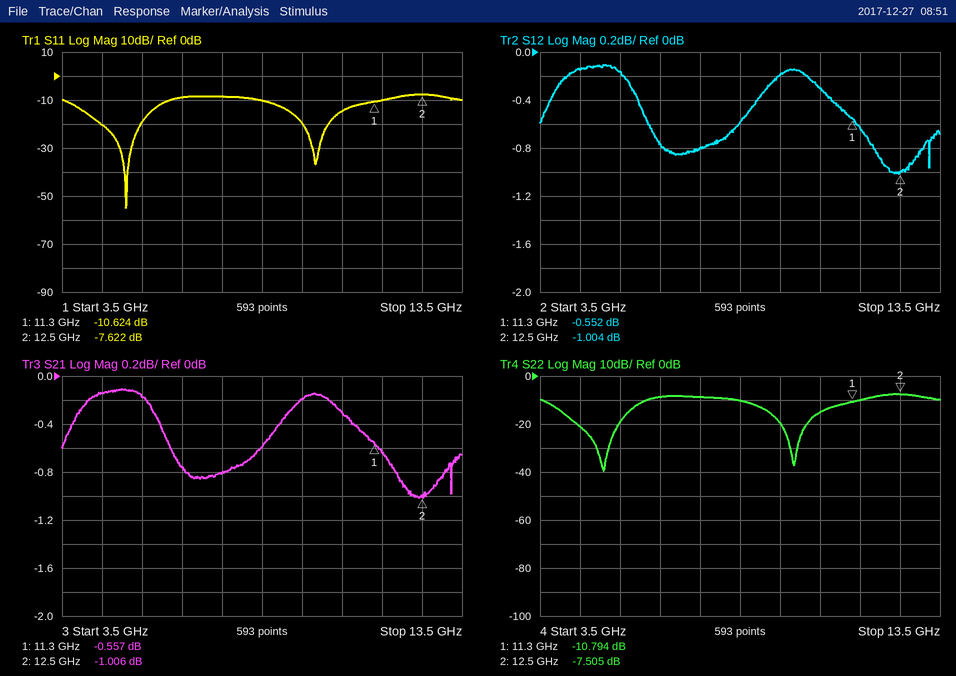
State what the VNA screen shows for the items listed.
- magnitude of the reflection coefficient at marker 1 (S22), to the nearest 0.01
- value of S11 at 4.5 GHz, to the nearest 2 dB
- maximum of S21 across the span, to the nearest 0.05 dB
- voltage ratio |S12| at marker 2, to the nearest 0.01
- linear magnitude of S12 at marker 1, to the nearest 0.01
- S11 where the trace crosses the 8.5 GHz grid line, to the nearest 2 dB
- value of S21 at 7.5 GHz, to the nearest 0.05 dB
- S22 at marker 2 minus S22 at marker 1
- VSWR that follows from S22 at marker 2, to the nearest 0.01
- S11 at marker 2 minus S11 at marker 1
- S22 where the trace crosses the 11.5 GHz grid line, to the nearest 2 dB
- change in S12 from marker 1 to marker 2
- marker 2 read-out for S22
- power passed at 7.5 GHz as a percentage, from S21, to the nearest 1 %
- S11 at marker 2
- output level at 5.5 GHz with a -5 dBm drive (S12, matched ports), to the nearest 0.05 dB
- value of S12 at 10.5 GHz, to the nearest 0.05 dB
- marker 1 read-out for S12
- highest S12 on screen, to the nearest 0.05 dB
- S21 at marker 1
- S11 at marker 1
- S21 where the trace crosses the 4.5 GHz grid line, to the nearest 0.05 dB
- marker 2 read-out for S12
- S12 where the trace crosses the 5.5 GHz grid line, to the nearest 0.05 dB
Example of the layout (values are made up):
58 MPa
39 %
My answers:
0.29
-20 dB
-0.10 dB
0.89
0.94
-10 dB
-0.80 dB
3.289 dB
2.46
3.002 dB
-10 dB
-0.452 dB
-7.505 dB
83 %
-7.622 dB
-5.15 dBm
-0.30 dB
-0.552 dB
-0.10 dB
-0.557 dB
-10.624 dB
-0.15 dB
-1.004 dB
-0.15 dB
